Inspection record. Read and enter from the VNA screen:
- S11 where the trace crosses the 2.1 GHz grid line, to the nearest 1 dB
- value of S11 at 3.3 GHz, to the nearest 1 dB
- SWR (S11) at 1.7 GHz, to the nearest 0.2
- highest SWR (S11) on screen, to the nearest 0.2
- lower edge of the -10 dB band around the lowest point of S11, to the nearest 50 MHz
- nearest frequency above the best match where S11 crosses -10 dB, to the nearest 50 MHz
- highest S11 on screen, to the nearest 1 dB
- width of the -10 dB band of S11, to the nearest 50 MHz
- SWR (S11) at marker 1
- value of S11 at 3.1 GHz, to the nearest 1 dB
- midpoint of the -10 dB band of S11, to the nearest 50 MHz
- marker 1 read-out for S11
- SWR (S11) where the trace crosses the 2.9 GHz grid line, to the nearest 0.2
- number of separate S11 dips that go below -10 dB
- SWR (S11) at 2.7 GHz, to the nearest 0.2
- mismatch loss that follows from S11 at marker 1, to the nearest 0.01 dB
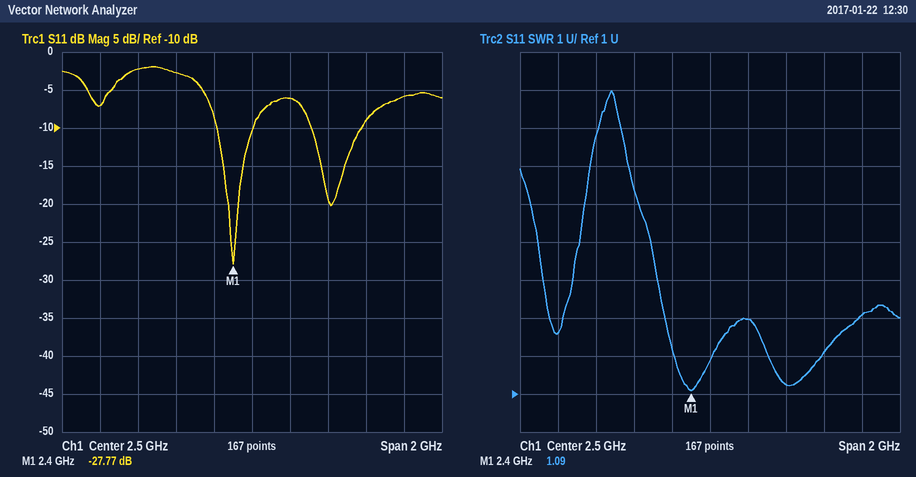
-3 dB
-6 dB
2.6
9.0
2.30 GHz
2.50 GHz
-2 dB
200 MHz
1.09
-9 dB
2.40 GHz
-27.77 dB
1.2
2
3.0
0.01 dB
